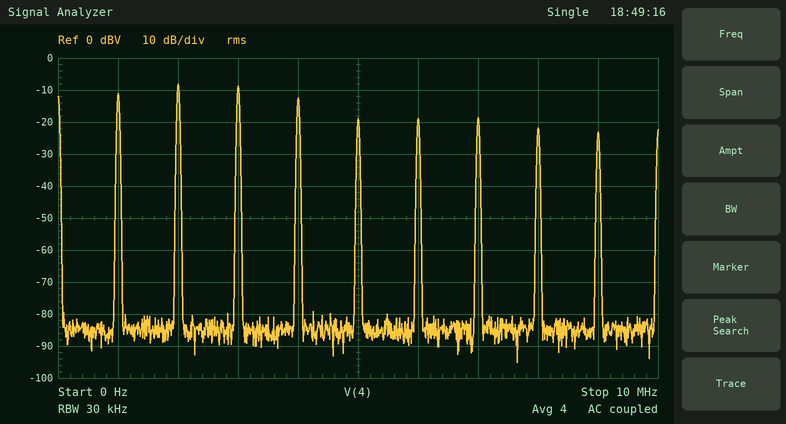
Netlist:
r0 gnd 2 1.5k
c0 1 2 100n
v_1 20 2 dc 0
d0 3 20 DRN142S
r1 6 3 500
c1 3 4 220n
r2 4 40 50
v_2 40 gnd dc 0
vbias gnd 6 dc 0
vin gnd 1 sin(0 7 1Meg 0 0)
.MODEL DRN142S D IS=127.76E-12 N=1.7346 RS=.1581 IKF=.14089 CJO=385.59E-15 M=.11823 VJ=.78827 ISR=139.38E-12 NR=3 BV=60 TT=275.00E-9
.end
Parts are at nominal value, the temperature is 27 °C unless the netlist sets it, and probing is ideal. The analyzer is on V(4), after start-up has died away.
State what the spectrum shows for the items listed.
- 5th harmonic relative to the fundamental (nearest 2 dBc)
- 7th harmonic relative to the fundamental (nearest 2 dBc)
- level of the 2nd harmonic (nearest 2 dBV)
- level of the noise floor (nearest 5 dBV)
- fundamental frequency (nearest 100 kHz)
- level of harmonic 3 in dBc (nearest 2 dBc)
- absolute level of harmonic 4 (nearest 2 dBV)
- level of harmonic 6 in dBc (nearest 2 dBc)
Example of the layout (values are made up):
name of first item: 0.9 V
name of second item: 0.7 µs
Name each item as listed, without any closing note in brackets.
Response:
5th harmonic relative to the fundamental: -8 dBc
7th harmonic relative to the fundamental: -8 dBc
level of the 2nd harmonic: -8 dBV
level of the noise floor: -85 dBV
fundamental frequency: 1.0 MHz
level of harmonic 3 in dBc: 2 dBc
absolute level of harmonic 4: -12 dBV
level of harmonic 6 in dBc: -8 dBc
